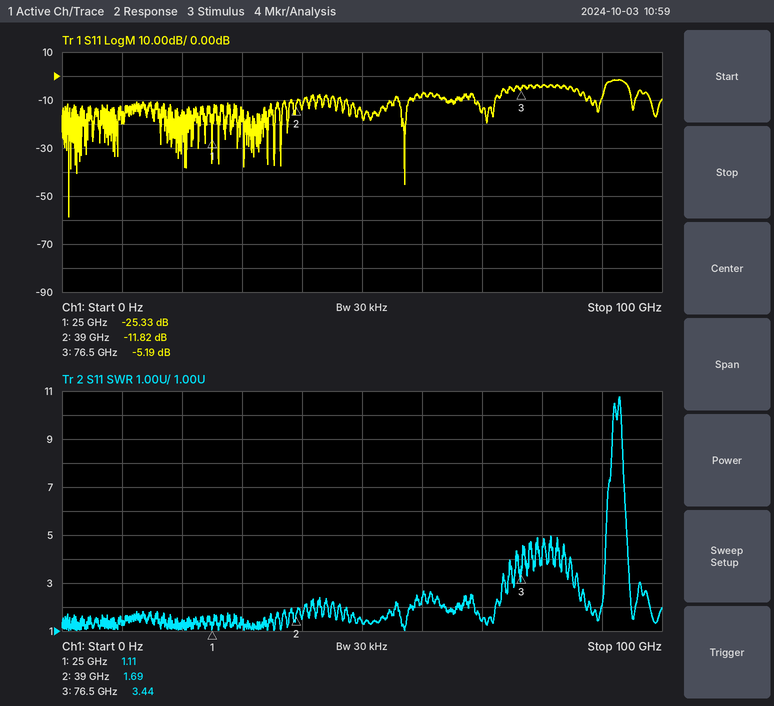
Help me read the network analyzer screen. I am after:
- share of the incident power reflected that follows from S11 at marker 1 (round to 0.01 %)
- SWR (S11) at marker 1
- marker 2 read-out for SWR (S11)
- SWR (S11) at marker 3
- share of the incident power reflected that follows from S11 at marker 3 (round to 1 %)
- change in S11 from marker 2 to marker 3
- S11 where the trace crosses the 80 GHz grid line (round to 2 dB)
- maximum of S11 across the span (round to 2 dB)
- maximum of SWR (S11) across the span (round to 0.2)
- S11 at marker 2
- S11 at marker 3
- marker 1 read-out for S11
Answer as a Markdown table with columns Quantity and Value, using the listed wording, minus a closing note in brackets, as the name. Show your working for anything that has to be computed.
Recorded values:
| Quantity | Value |
|---|---|
| share of the incident power reflected that follows from S11 at marker 1 | 10^(-25.33/10) ≈ 0.29 % |
| SWR (S11) at marker 1 | 1.11 |
| marker 2 read-out for SWR | 1.69 |
| SWR (S11) at marker 3 | 3.44 |
| share of the incident power reflected that follows from S11 at marker 3 | 10^(-5.19/10) ≈ 30 % |
| change in S11 from marker 2 to marker 3 | -5.19 − (-11.82) = 6.63 dB |
| S11 where the trace crosses the 80 GHz grid line | -4 dB |
| maximum of S11 across the span | -2 dB |
| maximum of SWR (S11) across the span | 10.8 |
| S11 at marker 2 | -11.82 dB |
| S11 at marker 3 | -5.19 dB |
| marker 1 read-out for S11 | -25.33 dB |
